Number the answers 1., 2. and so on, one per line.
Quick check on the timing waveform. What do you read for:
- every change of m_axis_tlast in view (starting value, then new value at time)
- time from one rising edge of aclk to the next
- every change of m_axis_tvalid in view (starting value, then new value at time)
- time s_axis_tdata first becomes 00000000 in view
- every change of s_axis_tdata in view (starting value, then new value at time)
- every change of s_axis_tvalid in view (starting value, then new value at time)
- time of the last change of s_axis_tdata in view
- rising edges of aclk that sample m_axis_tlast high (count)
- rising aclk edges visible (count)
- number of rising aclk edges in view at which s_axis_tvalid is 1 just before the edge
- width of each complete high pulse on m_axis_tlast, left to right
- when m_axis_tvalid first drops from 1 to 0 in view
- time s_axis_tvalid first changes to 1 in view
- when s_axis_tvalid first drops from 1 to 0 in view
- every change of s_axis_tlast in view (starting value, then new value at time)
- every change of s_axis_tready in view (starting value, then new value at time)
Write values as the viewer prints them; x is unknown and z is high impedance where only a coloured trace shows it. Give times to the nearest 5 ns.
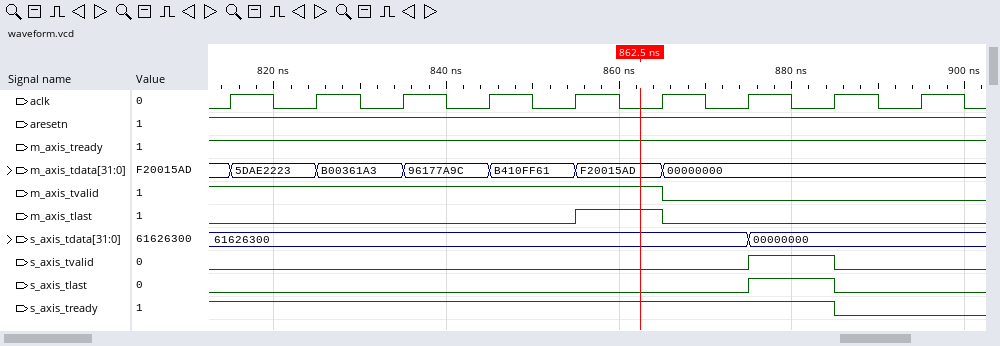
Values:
1. 0, 1 at 855 ns, 0 at 865 ns
2. 10 ns
3. 1, 0 at 865 ns
4. 875 ns
5. 61626300, 00000000 at 875 ns
6. 0, 1 at 875 ns, 0 at 885 ns
7. 875 ns
8. 1
9. 9
10. 1
11. 10 ns
12. 865 ns
13. 875 ns
14. 885 ns
15. 0, 1 at 875 ns, 0 at 885 ns
16. 1, 0 at 885 ns
